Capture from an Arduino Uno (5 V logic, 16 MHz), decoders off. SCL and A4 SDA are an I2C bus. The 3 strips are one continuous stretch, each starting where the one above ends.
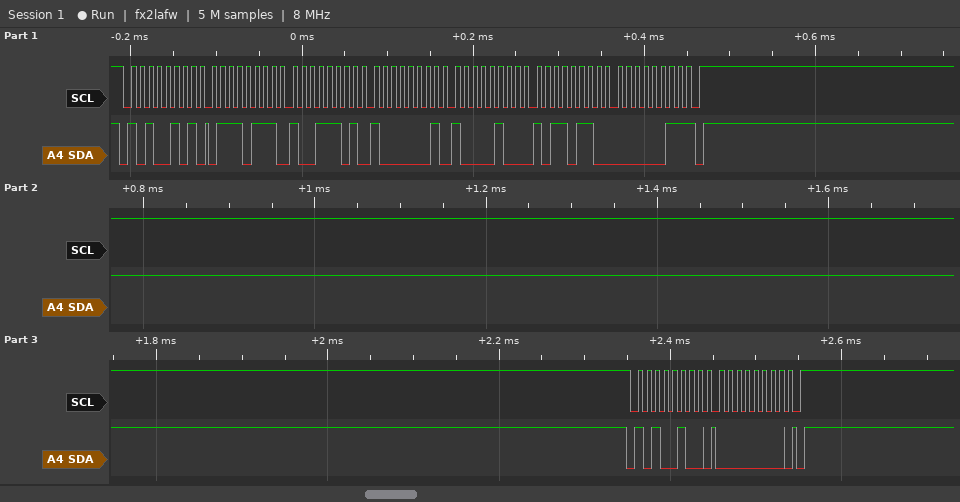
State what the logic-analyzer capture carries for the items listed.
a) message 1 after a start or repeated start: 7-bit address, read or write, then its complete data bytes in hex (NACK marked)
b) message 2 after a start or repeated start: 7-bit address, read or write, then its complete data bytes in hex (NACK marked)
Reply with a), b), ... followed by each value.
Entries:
a) 0x52 read: 77 9D 81 84 B6 03 NACK
b) 0x52 write: 00
